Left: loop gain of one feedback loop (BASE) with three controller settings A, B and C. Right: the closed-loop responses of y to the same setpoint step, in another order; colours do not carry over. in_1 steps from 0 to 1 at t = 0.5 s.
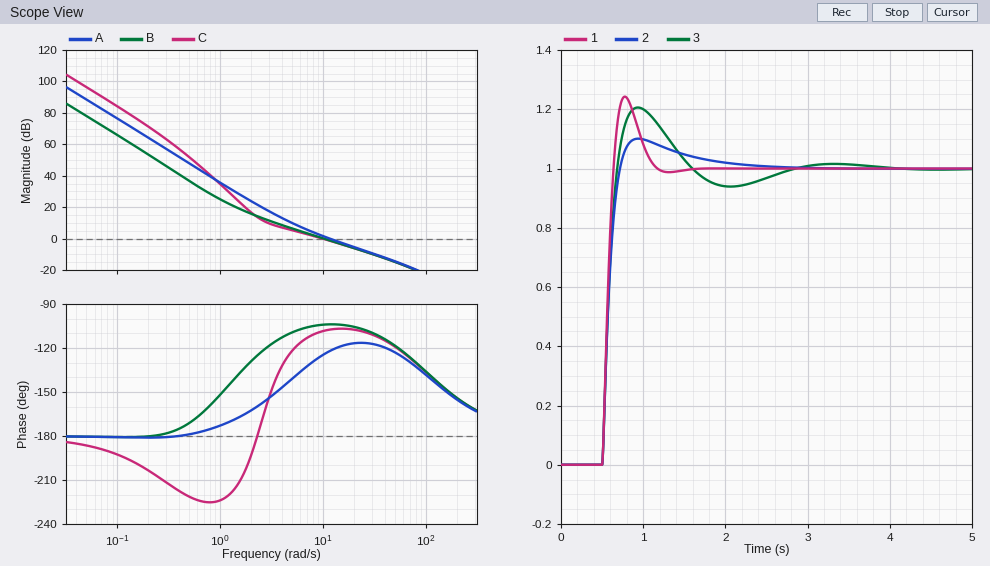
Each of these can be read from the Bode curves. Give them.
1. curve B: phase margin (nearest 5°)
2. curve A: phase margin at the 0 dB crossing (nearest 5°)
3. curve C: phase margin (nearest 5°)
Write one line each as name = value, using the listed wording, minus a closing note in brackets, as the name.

curve B: phase margin = 75°
curve A: phase margin at the 0 dB crossing = 60°
curve C: phase margin = 70°
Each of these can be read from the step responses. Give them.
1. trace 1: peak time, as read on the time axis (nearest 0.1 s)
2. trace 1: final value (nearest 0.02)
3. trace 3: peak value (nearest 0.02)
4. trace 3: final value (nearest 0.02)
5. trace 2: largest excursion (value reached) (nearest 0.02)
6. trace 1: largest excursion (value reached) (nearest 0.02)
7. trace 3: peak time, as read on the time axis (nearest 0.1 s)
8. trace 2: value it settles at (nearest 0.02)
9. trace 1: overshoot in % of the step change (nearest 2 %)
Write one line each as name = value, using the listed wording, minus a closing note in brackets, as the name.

trace 1: peak time, as read on the time axis = 0.8 s
trace 1: final value = 1.00
trace 3: peak value = 1.20
trace 3: final value = 1.00
trace 2: largest excursion (value reached) = 1.10
trace 1: largest excursion (value reached) = 1.24
trace 3: peak time, as read on the time axis = 0.9 s
trace 2: value it settles at = 1.00
trace 1: overshoot in % of the step change = 24 %
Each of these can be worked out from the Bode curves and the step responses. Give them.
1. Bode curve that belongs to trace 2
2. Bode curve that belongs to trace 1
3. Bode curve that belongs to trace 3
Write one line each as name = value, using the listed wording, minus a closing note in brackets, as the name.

Bode curve that belongs to trace 2 = B
Bode curve that belongs to trace 1 = A
Bode curve that belongs to trace 3 = C
